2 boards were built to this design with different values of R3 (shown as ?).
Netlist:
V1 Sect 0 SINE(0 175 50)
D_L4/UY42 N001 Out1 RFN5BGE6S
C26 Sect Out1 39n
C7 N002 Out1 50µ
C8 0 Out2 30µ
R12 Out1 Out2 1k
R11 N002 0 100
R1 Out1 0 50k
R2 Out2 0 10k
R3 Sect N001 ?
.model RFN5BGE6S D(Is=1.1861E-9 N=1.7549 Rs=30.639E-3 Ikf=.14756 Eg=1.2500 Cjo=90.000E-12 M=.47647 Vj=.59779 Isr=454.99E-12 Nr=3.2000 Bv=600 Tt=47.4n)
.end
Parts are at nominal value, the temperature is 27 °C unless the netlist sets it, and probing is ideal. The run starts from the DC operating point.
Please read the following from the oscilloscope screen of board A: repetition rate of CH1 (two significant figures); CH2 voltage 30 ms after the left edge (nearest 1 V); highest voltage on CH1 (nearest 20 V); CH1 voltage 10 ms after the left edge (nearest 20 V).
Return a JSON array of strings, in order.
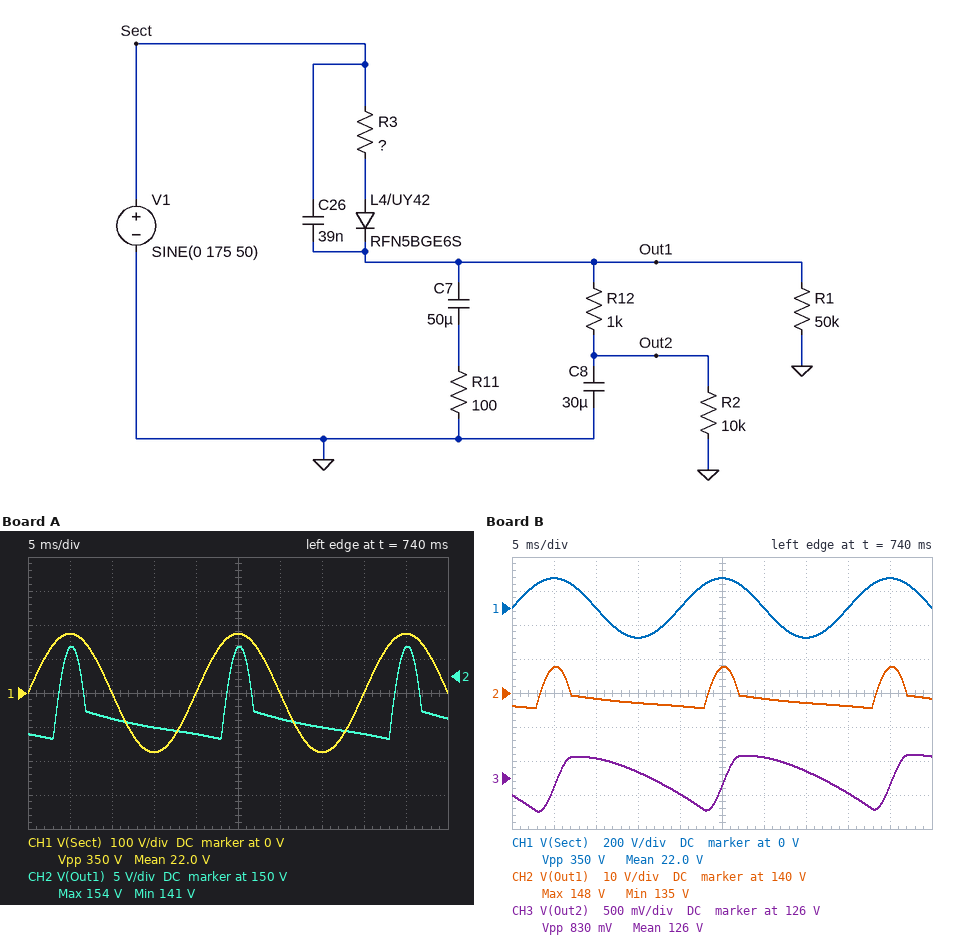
["50 Hz", "144 V", "180 V", "0 V"]
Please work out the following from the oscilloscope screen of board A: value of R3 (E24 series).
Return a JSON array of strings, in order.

["160 Ω"]
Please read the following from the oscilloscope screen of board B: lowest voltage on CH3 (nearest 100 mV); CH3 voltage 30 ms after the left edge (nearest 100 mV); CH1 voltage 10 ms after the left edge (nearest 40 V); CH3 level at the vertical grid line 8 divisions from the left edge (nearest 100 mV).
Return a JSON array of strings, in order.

["125.5 V", "126.3 V", "0 V", "125.8 V"]
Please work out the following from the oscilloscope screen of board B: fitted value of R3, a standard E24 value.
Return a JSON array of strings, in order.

["240 Ω"]
